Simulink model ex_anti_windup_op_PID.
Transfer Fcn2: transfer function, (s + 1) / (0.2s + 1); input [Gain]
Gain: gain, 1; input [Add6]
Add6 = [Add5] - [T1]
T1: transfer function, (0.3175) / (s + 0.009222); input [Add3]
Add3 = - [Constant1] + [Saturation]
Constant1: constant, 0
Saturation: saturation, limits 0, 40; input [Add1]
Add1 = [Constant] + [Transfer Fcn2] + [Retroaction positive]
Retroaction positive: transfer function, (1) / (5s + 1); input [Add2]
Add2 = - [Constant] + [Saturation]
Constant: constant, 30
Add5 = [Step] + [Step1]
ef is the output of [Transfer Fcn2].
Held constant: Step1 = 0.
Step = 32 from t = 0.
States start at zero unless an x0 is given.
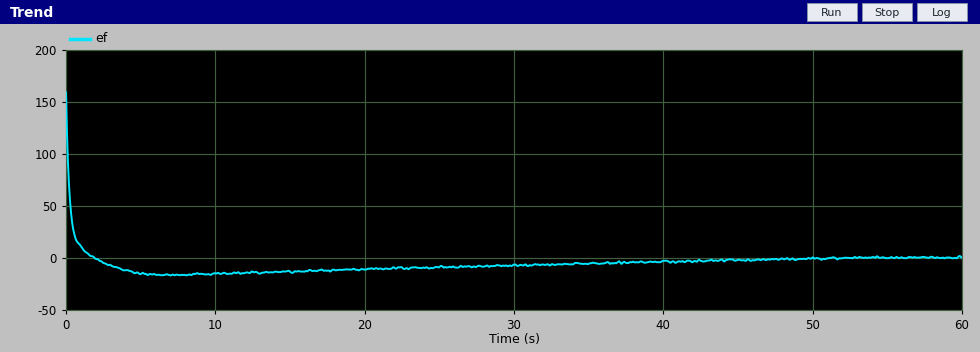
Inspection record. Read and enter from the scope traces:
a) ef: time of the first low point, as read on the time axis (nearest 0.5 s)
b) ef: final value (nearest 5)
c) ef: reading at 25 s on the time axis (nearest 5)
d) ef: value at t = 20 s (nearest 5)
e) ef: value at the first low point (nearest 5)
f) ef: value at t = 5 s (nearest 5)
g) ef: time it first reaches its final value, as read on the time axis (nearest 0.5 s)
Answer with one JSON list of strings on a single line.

["7.0 s", "0", "-10", "-10", "-15", "-15", "2.0 s"]
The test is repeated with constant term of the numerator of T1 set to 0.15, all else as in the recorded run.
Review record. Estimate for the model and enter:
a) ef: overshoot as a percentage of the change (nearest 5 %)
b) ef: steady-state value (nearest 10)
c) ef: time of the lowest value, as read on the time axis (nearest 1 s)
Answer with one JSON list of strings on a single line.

["10 %", "0", "12 s"]
